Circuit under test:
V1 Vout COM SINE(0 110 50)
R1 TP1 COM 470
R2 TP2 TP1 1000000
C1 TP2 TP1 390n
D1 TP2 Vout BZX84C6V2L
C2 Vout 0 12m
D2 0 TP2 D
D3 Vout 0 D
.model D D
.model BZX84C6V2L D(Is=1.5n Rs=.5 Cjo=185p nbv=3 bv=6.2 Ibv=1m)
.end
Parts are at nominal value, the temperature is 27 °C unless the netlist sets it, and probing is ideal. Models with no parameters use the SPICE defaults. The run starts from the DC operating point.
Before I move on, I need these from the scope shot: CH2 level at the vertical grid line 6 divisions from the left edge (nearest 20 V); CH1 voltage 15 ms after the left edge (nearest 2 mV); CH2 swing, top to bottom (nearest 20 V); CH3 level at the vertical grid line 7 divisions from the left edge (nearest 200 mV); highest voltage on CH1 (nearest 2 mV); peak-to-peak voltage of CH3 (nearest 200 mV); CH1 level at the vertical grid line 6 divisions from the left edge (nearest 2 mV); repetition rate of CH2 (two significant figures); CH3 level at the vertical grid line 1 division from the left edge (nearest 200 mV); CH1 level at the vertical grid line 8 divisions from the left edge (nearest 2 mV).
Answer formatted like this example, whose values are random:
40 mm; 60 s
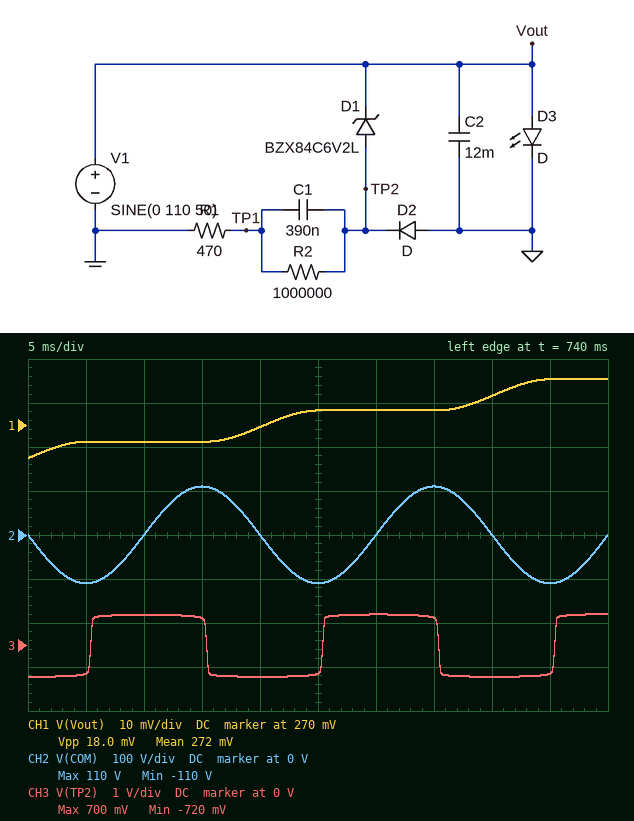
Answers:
0 V; 266 mV; 220 V; 600 mV; 280 mV; 1.4 V; 274 mV; 50 Hz; -600 mV; 276 mV
